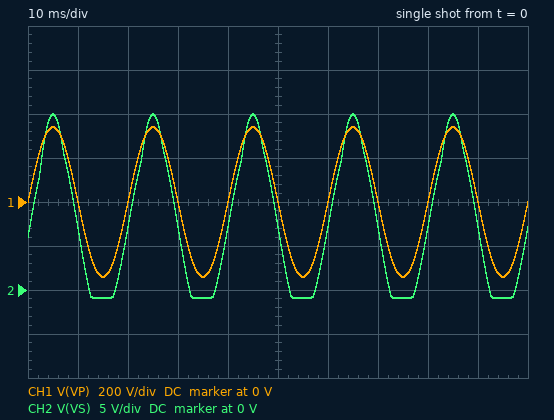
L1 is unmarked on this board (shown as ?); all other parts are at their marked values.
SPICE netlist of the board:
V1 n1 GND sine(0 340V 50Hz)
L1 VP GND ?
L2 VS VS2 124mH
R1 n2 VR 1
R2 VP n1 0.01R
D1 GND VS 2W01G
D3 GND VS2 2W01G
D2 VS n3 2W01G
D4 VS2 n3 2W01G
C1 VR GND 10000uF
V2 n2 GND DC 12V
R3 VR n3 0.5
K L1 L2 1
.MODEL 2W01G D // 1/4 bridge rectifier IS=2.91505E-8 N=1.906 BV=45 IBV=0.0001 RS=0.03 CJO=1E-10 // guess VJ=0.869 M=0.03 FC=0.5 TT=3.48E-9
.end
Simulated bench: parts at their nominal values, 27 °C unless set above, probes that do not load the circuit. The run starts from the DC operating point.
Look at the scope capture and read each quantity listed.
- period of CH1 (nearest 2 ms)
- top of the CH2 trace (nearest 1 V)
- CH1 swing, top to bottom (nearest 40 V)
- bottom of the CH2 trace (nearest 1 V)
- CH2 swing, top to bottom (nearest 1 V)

20 ms
20 V
680 V
-1 V
21 V
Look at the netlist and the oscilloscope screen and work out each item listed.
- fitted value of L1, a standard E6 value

33 H
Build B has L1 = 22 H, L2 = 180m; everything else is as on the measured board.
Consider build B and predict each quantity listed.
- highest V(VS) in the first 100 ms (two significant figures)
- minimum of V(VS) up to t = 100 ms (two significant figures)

30 V
-910 mV
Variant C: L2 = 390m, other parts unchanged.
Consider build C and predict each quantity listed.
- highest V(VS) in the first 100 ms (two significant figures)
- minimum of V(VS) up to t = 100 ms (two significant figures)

36 V
-920 mV
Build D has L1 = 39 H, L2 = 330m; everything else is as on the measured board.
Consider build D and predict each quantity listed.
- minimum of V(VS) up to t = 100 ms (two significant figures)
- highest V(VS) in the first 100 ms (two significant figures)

-910 mV
30 V
